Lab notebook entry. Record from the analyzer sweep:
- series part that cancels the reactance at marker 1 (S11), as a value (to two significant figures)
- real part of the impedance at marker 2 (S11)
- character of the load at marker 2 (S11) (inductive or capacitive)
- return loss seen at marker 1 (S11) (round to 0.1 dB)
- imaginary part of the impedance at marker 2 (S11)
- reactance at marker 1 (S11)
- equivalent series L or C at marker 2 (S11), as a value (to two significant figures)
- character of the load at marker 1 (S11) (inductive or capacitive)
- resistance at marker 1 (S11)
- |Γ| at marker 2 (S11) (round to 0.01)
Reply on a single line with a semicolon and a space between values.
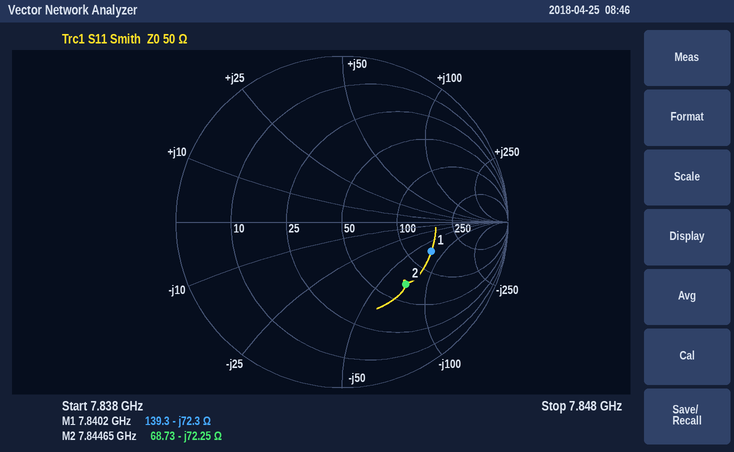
1.5 nH; 68.73 Ω; capacitive; 4.9 dB; -72.25 Ω; -72.3 Ω; 280 fF; capacitive; 139.3 Ω; 0.54
